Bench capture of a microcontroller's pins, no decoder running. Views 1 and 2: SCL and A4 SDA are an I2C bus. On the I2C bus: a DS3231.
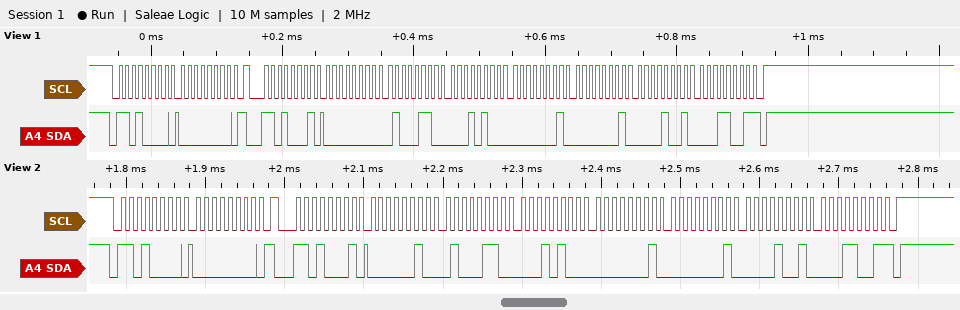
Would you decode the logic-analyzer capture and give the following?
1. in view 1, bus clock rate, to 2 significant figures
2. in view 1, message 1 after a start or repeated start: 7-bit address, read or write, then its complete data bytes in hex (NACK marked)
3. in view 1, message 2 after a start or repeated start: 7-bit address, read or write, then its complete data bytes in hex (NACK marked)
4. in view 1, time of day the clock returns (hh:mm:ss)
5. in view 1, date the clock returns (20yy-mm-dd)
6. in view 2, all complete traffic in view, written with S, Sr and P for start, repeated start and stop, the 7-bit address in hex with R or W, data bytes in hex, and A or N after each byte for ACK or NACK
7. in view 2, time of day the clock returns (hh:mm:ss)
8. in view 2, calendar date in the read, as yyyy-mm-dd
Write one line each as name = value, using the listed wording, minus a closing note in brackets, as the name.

in view 1, bus clock rate, to 2 significant figures = 100 kHz
in view 1, message 1 after a start or repeated start: 7-bit address, read or write, then its complete data bytes in hex = 0x68 write: 00
in view 1, message 2 after a start or repeated start: 7-bit address, read or write, then its complete data bytes in hex = 0x68 read: 00 46 14 01 01 09 19 NACK
in view 1, time of day the clock returns = 14:46:00
in view 1, date the clock returns = 2019-09-01
in view 2, all complete traffic in view, written with S, Sr and P for start, repeated start and stop, the 7-bit address in hex with R or W, data bytes in hex, and A or N after each byte for ACK or NACK = S 68W A 00 A Sr 68R A 02 A 46 A 14 A 01 A 01 A 09 A 19 N P
in view 2, time of day the clock returns = 14:46:02
in view 2, calendar date in the read, as yyyy-mm-dd = 2019-09-01
